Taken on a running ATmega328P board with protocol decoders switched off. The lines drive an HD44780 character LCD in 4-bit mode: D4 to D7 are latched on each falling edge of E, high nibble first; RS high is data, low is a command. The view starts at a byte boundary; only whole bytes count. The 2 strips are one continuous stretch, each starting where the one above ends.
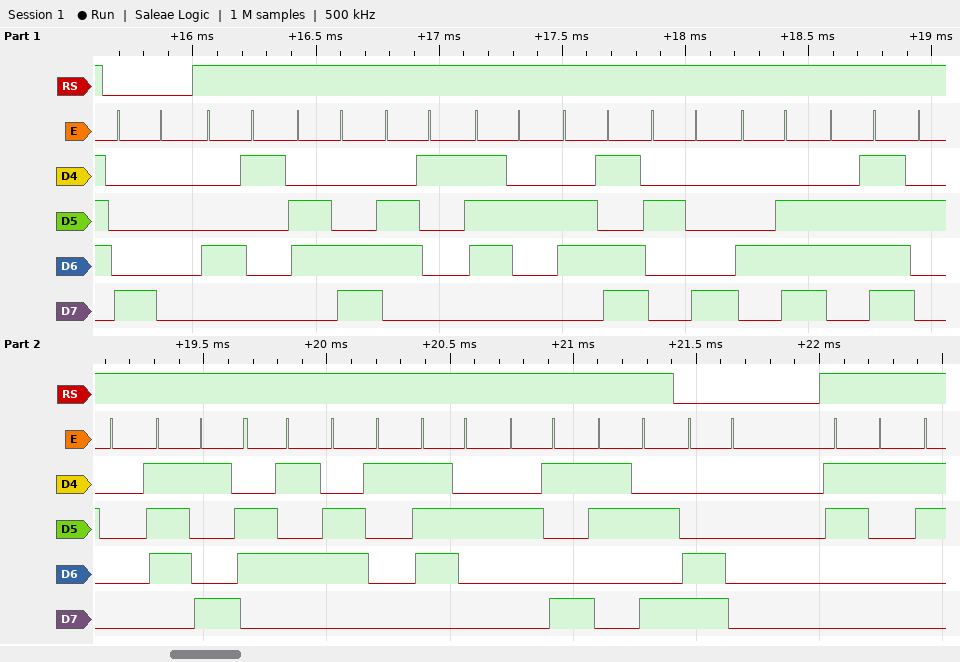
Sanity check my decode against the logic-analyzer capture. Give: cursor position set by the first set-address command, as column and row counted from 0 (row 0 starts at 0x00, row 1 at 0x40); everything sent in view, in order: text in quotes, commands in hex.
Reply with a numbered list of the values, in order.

1. column 0, row 0
2. 0x80 "Alarm(No year):" 0xC0 "1"
